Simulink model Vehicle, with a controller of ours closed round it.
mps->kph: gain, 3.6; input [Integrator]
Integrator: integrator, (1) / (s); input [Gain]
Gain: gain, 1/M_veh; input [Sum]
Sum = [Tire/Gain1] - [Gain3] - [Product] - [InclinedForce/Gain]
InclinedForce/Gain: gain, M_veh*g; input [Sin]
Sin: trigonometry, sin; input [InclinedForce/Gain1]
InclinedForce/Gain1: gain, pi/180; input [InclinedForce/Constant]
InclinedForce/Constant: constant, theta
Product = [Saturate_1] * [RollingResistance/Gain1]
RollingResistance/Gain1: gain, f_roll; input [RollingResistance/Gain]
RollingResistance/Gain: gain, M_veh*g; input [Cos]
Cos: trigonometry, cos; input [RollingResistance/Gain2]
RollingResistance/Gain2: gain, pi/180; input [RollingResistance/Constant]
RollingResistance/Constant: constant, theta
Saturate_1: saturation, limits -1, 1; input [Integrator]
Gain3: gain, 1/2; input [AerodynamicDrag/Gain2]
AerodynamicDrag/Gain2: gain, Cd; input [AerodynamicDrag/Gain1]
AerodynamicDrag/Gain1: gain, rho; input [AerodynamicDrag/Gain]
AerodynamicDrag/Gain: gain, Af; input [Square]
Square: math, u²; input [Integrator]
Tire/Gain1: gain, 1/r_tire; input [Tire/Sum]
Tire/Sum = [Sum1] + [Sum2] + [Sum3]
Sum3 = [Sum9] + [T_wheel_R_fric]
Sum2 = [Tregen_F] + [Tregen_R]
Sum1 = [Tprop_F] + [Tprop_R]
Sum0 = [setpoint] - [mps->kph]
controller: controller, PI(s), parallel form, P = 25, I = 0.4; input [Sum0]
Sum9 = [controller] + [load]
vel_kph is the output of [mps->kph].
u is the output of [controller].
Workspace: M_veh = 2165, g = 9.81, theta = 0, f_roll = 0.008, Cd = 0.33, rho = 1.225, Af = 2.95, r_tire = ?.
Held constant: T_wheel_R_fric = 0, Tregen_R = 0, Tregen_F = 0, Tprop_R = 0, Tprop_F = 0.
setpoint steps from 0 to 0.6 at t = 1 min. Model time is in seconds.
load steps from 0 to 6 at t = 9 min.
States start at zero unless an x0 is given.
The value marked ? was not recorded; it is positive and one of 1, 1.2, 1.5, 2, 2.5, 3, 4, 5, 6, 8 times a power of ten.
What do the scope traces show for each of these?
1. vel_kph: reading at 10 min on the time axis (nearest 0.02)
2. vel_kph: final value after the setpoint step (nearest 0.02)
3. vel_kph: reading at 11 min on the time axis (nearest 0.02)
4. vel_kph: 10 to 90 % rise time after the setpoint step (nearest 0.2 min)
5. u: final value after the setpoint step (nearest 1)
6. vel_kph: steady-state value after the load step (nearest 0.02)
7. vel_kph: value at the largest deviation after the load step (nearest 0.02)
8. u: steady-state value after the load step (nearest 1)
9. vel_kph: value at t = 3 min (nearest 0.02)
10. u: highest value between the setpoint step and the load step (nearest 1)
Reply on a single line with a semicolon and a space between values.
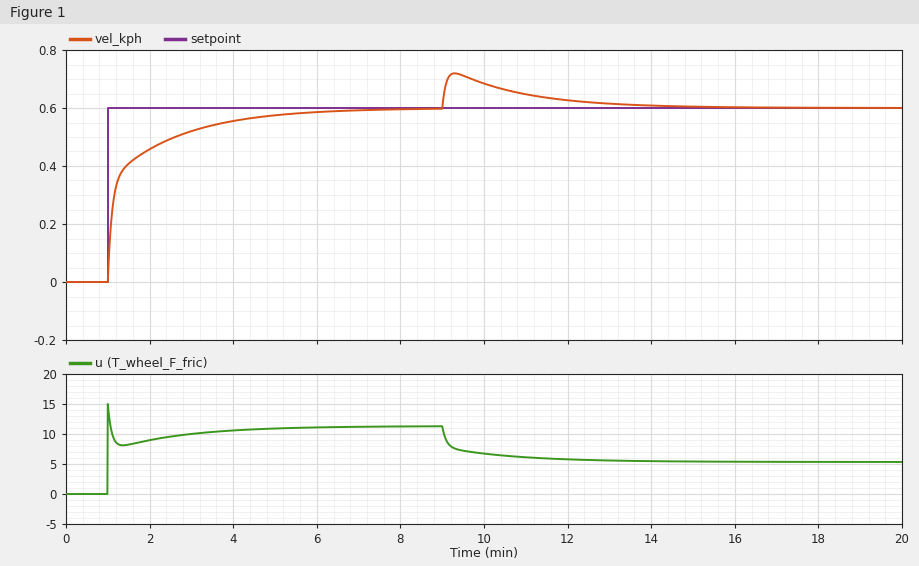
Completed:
0.68; 0.60; 0.64; 2.4 min; 11; 0.60; 0.72; 5; 0.52; 15
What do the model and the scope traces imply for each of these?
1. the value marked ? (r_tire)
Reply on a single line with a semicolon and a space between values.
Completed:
0.4
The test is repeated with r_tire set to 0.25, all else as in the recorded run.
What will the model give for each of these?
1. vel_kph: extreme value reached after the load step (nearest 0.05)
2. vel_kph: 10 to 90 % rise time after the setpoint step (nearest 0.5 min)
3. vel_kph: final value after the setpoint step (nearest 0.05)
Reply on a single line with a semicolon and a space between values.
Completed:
0.75; 1.5 min; 0.60
